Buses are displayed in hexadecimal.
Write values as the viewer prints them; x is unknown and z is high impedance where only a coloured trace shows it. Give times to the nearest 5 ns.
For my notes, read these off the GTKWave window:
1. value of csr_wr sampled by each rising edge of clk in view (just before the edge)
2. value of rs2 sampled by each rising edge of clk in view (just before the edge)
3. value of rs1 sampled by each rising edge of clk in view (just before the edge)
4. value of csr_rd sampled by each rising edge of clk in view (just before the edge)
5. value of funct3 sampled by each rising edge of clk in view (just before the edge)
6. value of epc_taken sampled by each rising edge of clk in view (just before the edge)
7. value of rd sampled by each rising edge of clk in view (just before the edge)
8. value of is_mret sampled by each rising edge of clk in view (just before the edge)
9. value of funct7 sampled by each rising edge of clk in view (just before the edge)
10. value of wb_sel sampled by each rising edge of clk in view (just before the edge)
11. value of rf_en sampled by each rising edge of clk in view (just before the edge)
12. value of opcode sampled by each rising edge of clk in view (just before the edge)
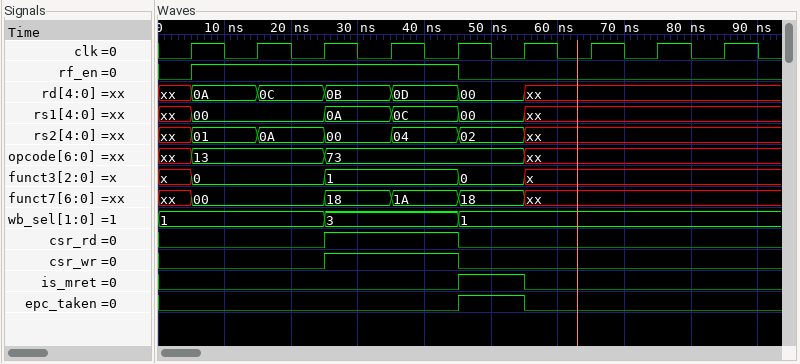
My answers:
0 0 0 1 1 0 0 0 0
xx, 01, 0A, 00, 04, 02, xx, xx, xx
xx, 00, 00, 0A, 0C, 00, xx, xx, xx
0 0 0 1 1 0 0 0 0
x, 0, 0, 1, 1, 0, x, x, x
0 0 0 0 0 1 0 0 0
xx, 0A, 0C, 0B, 0D, 00, xx, xx, xx
0 0 0 0 0 1 0 0 0
xx, 00, 00, 18, 1A, 18, xx, xx, xx
1, 1, 1, 3, 3, 1, 1, 1, 1
0 1 1 1 1 0 0 0 0
xx, 13, 13, 73, 73, 73, xx, xx, xx
